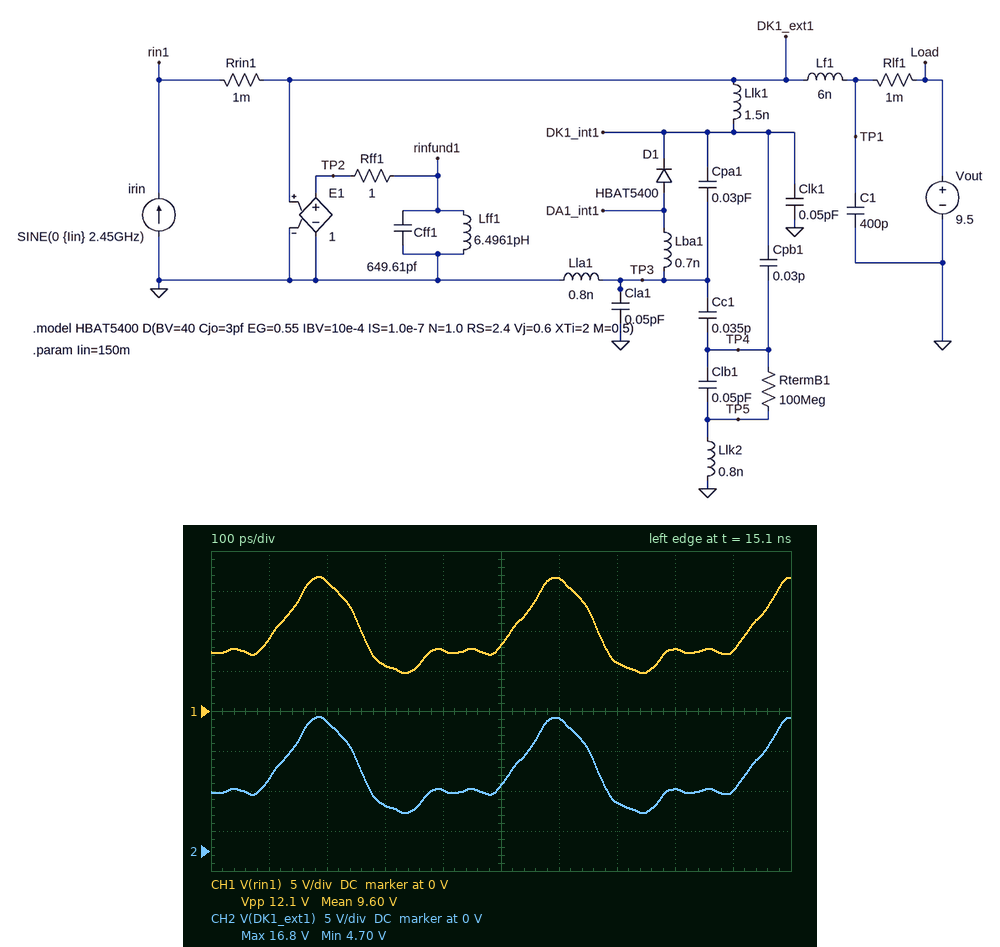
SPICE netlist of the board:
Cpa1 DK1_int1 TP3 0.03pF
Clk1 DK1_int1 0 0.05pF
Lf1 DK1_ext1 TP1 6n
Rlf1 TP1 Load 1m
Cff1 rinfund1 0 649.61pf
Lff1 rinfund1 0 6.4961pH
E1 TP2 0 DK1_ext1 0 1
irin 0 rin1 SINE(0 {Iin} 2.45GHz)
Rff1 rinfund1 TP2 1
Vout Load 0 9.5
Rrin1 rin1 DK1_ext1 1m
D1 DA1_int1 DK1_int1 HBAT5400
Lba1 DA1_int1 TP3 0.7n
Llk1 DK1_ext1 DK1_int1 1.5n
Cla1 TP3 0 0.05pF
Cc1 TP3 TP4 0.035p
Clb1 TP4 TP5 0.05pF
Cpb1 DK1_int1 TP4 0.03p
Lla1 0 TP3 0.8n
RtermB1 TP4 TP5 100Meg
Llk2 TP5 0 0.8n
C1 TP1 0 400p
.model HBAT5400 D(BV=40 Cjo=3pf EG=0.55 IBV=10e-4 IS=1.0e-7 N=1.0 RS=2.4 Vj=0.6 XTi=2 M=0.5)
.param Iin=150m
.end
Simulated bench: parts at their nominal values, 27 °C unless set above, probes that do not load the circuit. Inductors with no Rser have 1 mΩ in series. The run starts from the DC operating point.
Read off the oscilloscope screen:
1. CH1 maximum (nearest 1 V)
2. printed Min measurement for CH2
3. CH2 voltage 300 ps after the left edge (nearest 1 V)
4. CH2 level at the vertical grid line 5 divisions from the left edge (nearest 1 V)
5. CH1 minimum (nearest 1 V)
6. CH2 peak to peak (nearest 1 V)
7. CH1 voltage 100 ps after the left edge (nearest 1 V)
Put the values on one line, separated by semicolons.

17 V; 4.70 V; 6 V; 8 V; 5 V; 12 V; 9 V
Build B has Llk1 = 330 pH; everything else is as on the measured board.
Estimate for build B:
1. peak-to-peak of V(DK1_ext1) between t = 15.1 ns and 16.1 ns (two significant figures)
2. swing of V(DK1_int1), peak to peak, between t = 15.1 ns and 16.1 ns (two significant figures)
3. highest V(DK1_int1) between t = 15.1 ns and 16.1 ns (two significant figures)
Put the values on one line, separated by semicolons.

20 V; 22 V; 23 V
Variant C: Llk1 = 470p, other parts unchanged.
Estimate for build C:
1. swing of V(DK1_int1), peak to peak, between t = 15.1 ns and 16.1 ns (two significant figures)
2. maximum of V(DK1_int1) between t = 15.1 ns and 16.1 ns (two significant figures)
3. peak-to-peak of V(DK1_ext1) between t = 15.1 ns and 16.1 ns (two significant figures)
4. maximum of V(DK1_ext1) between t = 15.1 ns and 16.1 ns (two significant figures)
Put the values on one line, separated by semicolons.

22 V; 23 V; 19 V; 21 V
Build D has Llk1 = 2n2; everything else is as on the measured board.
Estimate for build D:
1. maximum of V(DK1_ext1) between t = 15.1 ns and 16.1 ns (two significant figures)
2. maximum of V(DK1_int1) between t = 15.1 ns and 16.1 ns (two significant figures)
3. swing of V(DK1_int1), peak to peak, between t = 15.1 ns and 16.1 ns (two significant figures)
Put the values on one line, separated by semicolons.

14 V; 21 V; 18 V
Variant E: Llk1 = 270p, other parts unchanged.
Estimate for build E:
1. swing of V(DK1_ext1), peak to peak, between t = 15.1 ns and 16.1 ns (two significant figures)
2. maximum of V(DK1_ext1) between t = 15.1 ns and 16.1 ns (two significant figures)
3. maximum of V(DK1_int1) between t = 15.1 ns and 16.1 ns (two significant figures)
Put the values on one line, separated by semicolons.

21 V; 22 V; 23 V
